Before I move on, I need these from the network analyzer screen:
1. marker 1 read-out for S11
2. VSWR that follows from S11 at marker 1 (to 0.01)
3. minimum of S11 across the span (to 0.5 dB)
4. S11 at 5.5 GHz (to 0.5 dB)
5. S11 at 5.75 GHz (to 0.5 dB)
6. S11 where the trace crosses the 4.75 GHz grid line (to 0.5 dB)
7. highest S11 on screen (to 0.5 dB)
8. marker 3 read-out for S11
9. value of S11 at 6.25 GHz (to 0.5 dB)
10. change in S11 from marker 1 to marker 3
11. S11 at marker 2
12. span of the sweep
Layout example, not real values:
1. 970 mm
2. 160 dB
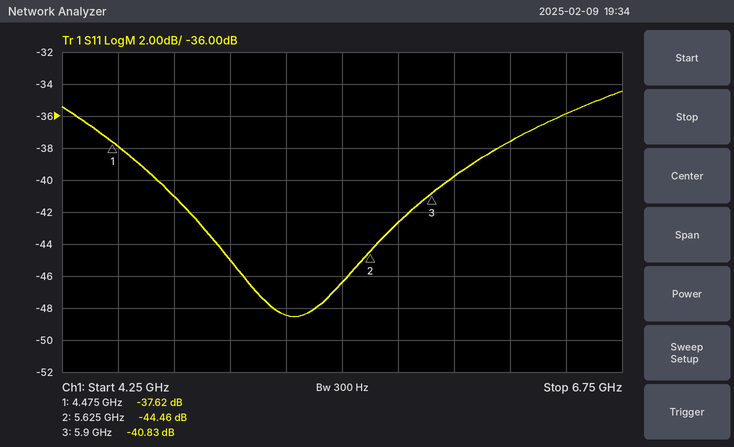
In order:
1. -37.62 dB
2. 1.03
3. -48.5 dB
4. -46.5 dB
5. -42.5 dB
6. -41.0 dB
7. -34.5 dB
8. -40.83 dB
9. -37.5 dB
10. -3.21 dB
11. -44.46 dB
12. 2.5 GHz
